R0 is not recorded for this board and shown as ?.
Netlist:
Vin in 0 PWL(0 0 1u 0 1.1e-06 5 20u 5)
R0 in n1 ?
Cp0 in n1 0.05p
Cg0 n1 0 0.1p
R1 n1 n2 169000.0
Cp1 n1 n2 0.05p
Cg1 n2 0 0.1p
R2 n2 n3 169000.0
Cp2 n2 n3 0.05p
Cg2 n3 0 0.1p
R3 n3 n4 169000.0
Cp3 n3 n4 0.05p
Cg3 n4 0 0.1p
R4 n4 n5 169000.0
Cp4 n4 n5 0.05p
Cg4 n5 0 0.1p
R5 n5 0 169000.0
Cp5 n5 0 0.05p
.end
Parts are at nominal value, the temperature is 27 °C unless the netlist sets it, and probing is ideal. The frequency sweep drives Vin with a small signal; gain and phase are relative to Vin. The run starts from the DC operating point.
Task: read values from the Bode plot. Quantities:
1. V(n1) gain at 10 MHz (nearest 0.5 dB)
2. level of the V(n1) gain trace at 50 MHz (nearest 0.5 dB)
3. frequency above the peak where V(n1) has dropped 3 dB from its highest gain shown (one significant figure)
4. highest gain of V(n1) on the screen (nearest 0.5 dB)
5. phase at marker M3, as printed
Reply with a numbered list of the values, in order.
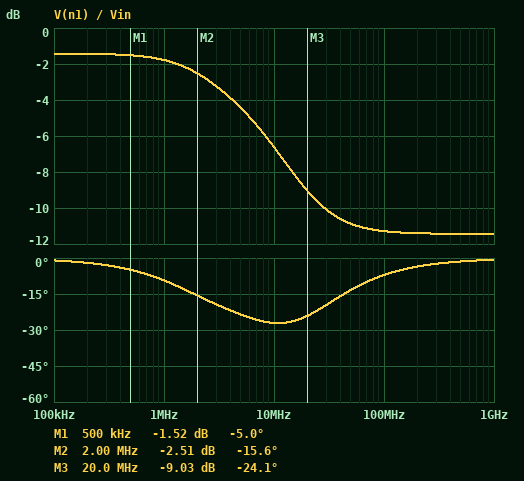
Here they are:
1. -6.5 dB
2. -11.0 dB
3. 5 MHz
4. -1.5 dB
5. -24.1 deg
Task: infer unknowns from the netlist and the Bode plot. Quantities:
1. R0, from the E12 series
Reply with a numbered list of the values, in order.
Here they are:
1. 150 kΩ
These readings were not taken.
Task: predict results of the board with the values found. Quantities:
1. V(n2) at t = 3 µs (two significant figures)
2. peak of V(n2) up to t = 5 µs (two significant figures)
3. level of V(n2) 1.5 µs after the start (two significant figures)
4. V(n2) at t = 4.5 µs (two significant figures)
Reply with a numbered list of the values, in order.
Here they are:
1. 3.4 V
2. 3.4 V
3. 3.4 V
4. 3.4 V
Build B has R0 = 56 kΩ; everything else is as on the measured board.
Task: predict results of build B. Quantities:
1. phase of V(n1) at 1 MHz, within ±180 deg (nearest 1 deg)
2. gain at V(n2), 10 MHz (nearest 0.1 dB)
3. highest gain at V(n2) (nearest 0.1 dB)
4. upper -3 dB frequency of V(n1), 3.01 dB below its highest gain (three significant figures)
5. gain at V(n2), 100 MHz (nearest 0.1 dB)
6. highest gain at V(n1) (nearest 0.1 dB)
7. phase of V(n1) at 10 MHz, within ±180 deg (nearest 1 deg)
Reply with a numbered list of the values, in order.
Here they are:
1. -4 deg
2. -9.7 dB
3. -2.5 dB
4. 15.1 MHz
5. -21.7 dB
6. -0.6 dB
7. -21 deg
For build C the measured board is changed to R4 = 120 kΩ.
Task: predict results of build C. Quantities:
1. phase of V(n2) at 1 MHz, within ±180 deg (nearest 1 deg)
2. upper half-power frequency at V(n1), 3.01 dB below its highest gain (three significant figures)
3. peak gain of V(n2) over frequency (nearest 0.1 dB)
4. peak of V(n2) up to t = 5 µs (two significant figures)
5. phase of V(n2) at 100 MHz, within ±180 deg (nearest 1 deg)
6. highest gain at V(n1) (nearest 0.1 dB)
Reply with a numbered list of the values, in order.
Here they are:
1. -17 deg
2. 5.14 MHz
3. -3.6 dB
4. 3.3 V
5. -13 deg
6. -1.5 dB
